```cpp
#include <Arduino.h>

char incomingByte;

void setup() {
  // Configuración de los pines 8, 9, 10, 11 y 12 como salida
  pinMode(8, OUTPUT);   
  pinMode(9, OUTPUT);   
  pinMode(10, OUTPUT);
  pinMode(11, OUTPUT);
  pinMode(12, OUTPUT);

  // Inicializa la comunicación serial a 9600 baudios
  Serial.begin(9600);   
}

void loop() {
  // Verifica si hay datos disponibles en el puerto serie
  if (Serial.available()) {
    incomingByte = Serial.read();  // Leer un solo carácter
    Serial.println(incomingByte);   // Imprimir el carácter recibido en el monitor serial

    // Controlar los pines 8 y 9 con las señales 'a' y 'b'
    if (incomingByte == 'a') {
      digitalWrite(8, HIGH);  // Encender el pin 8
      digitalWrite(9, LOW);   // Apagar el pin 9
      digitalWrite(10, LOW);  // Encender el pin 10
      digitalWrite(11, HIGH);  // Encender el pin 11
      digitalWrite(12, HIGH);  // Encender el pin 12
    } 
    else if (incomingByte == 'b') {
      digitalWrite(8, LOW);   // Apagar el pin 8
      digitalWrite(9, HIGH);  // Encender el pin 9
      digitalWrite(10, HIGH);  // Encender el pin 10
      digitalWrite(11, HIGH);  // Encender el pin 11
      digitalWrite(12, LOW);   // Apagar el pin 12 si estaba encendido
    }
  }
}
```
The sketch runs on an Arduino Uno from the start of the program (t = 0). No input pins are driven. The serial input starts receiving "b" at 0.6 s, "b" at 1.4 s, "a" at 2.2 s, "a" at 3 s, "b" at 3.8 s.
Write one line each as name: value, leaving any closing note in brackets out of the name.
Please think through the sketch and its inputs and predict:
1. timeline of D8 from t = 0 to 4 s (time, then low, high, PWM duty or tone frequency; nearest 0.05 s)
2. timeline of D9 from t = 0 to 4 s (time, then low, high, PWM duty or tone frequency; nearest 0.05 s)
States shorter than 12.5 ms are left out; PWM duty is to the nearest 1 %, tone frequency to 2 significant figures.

timeline of D8 from t = 0 to 4 s: 0 s low; 2.2 s high; 3.8 s low
timeline of D9 from t = 0 to 4 s: 0 s low; 0.6 s high; 2.2 s low; 3.8 s high
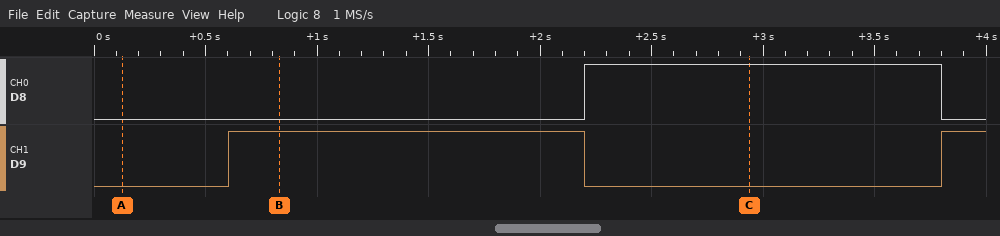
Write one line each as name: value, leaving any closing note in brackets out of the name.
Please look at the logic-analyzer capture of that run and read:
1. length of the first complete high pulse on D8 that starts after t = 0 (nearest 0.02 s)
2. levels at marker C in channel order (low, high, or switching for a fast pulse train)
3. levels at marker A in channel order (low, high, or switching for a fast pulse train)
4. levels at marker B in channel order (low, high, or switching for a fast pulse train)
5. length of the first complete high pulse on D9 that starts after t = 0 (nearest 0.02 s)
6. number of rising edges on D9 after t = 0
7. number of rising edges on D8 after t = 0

length of the first complete high pulse on D8 that starts after t = 0: 1.60 s
levels at marker C in channel order: D8 high, D9 low
levels at marker A in channel order: D8 low, D9 low
levels at marker B in channel order: D8 low, D9 high
length of the first complete high pulse on D9 that starts after t = 0: 1.60 s
number of rising edges on D9 after t = 0: 2
number of rising edges on D8 after t = 0: 1
